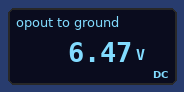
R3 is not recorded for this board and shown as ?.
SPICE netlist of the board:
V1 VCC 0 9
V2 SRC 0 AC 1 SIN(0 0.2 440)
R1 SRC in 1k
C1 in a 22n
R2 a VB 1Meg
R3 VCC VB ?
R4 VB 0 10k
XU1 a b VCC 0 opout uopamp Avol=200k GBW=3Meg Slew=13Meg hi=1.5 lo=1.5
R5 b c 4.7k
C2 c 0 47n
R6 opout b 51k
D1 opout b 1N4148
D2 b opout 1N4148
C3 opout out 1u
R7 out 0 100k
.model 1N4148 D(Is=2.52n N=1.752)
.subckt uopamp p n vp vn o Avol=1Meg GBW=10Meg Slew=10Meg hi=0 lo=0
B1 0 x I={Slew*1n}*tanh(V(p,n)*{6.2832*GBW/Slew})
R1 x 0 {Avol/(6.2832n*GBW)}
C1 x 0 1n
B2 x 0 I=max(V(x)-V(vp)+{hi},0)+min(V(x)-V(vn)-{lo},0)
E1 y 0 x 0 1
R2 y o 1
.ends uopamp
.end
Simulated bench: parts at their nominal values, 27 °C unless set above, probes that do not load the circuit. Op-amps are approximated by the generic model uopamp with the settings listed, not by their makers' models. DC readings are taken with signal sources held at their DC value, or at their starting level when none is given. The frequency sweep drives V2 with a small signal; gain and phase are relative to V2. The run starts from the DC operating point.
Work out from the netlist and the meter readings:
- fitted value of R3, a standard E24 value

3.9 kΩ
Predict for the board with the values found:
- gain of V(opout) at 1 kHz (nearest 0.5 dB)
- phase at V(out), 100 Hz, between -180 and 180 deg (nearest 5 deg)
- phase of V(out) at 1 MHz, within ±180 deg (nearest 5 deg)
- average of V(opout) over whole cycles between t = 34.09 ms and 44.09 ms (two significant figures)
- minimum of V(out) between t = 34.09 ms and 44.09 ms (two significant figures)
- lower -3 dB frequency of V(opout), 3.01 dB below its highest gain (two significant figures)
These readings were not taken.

19.5 dB
55 deg
-75 deg
6.5 V
-560 mV
710 Hz
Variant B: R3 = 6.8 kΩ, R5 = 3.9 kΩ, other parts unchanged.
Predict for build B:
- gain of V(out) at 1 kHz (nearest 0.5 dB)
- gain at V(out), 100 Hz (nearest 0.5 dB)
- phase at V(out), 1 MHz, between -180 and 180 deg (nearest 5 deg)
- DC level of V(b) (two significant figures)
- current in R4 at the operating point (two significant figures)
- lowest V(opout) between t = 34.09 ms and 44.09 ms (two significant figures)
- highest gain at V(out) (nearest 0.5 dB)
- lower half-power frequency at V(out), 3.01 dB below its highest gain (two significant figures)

20.5 dB
5.5 dB
-80 deg
5.4 V
540 µA
4.8 V
23.0 dB
860 Hz
